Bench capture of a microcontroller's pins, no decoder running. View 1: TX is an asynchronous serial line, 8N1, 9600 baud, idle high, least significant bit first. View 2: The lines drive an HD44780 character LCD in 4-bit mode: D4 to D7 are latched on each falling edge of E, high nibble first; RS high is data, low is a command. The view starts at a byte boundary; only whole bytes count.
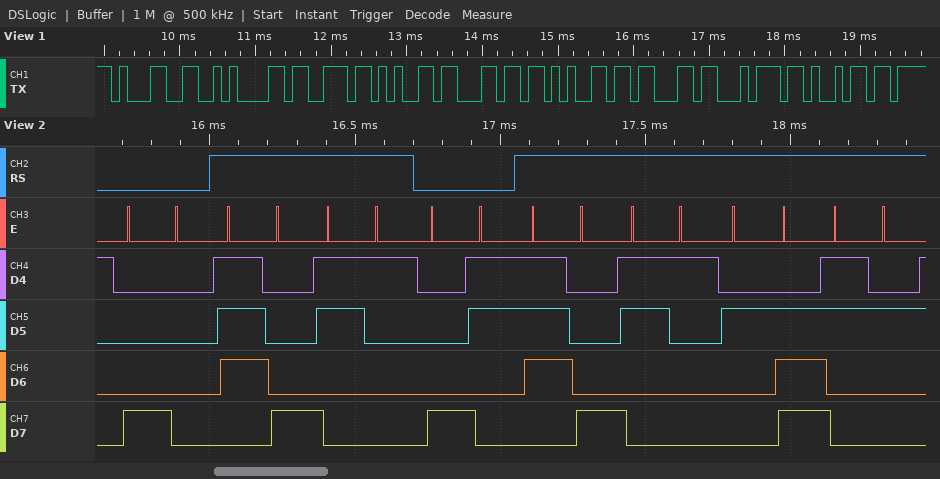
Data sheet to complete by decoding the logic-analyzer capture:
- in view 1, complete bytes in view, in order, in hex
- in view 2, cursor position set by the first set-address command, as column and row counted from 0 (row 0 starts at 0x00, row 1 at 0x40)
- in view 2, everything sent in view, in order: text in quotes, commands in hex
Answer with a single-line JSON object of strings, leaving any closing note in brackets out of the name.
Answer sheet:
{"in view 1, complete bytes in view, in order, in hex": "31 0A 73 65 6C 65 63 74 69", "in view 2, cursor position set by the first set-address command, as column and row counted from 0": "column 0, row 0", "in view 2, everything sent in view, in order: text in quotes, commands in hex": "0x80 \"x1\" 0x83 \"x1.2\""}
